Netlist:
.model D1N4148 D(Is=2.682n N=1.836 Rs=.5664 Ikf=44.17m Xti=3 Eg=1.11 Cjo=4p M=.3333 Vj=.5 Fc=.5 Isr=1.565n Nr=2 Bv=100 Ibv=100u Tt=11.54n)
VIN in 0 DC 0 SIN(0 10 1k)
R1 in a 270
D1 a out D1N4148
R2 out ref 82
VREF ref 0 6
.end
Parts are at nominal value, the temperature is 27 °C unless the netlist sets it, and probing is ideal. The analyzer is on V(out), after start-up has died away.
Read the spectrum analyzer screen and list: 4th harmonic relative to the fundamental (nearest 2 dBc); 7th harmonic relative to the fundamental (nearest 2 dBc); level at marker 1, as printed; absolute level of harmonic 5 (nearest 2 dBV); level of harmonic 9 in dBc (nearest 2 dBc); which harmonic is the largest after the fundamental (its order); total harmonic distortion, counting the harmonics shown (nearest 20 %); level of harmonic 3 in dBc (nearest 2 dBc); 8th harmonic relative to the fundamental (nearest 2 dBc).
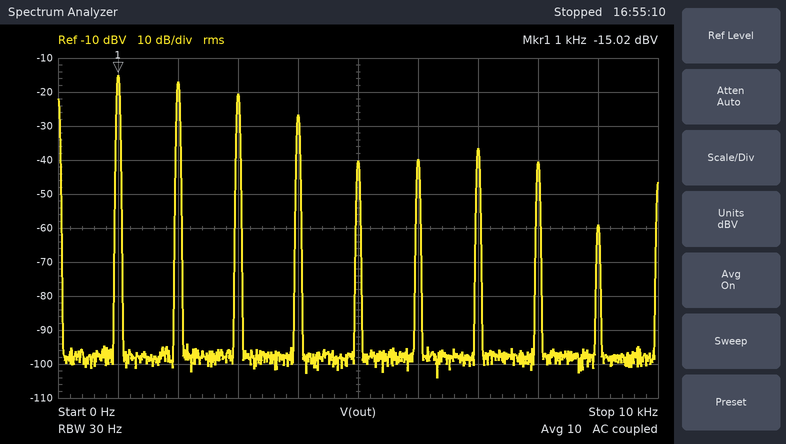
-12 dBc
-22 dBc
-15.02 dBV
-40 dBV
-44 dBc
2
100 %
-6 dBc
-26 dBc
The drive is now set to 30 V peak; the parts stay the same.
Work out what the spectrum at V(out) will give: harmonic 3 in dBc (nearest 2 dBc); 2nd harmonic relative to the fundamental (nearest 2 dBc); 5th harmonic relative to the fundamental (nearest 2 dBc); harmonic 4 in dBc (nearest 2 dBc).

-18 dBc
-6 dBc
-24 dBc
-22 dBc
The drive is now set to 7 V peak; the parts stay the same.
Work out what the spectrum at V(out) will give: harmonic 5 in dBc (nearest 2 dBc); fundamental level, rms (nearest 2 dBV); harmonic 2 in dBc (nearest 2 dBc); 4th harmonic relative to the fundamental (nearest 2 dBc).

-4 dBc
-40 dBV
0 dBc
-2 dBc
